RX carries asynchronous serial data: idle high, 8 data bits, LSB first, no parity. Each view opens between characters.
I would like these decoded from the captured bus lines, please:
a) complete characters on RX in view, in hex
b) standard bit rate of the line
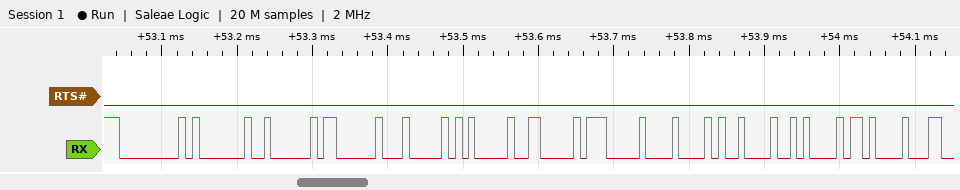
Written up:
00, 01, 02, 03, 04, 05, 06, 07, 08, 09, 0A, 0B
115200 baud
